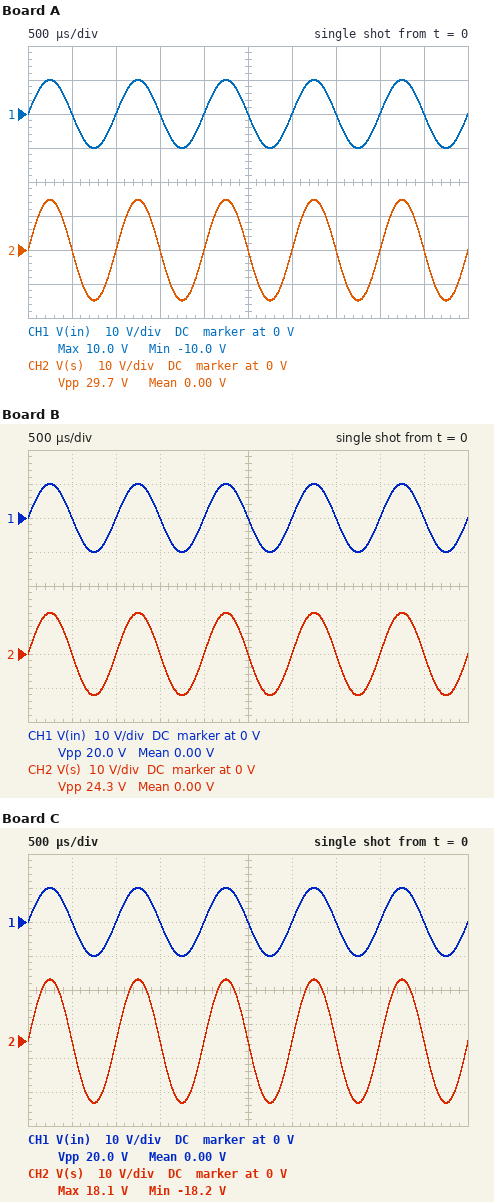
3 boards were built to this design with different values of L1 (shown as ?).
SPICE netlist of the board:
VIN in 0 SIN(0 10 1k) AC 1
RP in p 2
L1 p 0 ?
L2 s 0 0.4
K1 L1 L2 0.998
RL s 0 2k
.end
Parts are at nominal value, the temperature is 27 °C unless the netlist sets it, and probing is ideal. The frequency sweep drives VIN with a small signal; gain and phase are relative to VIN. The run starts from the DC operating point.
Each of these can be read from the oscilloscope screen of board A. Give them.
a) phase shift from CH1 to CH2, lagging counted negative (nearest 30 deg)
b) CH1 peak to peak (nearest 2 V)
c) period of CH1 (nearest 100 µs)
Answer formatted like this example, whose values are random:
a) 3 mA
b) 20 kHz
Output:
a) 0 deg
b) 20 V
c) 1.0 ms
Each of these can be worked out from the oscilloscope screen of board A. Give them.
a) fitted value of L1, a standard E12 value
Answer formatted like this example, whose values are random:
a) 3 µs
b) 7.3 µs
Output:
a) 180 mH
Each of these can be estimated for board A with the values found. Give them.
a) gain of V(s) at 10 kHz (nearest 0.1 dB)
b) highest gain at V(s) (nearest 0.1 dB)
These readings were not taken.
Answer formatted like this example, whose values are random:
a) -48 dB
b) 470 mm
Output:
a) 3.4 dB
b) 3.4 dB
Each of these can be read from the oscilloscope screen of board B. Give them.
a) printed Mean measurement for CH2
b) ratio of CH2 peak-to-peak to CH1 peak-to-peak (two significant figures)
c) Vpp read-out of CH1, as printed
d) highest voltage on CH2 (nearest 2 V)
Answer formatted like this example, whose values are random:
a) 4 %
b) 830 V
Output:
a) 0.00 V
b) 1.2
c) 20.0 V
d) 12 V
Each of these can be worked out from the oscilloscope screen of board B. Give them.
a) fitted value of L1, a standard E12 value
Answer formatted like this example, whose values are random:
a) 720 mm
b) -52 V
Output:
a) 270 mH
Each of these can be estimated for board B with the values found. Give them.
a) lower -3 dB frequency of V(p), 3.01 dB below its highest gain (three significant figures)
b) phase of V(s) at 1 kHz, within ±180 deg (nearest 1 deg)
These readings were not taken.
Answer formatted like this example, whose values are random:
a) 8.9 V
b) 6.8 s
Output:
a) 1.18 Hz
b) 0 deg
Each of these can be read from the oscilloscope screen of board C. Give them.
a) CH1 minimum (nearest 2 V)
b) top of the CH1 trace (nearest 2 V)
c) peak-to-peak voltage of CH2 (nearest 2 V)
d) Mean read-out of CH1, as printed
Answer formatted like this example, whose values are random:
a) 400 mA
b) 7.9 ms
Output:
a) -10 V
b) 10 V
c) 36 V
d) 0.00 V
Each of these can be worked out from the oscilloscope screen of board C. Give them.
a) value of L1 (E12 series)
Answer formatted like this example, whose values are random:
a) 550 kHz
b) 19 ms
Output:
a) 120 mH
